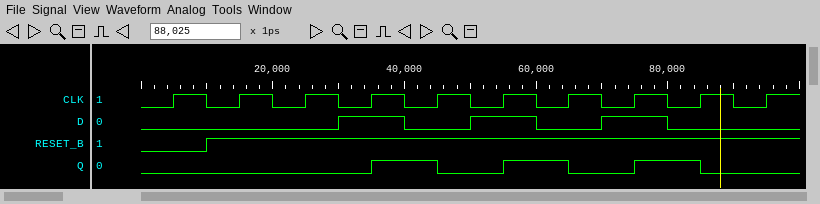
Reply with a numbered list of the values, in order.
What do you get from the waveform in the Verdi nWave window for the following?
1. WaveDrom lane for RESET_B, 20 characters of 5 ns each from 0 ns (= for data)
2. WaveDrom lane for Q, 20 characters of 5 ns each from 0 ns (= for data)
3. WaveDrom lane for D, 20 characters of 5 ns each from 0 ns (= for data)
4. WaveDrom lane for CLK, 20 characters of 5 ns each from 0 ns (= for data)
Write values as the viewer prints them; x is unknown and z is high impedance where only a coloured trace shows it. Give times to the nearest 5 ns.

1. {name: 'RESET_B', wave: '0.1.................'}
2. {name: 'Q', wave: '0......1.0.1.0.1.0..'}
3. {name: 'D', wave: '0.....1.0.1.0.1.0...'}
4. {name: 'CLK', wave: '01010101010101010101'}
